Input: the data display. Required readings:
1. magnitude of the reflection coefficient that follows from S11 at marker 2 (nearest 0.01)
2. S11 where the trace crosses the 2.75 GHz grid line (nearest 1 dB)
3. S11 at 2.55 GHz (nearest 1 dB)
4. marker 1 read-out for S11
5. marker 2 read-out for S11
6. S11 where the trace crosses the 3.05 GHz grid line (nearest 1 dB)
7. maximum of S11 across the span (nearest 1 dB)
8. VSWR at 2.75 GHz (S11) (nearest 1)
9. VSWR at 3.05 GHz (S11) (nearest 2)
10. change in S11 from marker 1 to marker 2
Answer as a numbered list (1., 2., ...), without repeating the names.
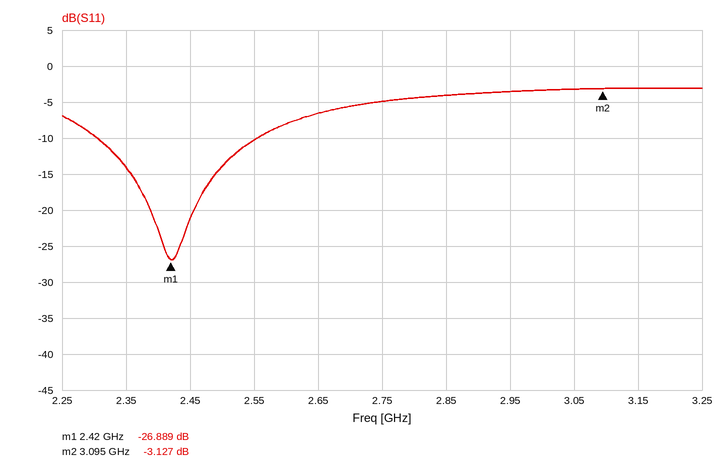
1. 0.70
2. -5 dB
3. -10 dB
4. -26.889 dB
5. -3.127 dB
6. -3 dB
7. -3 dB
8. 4
9. 6
10. 23.762 dB
